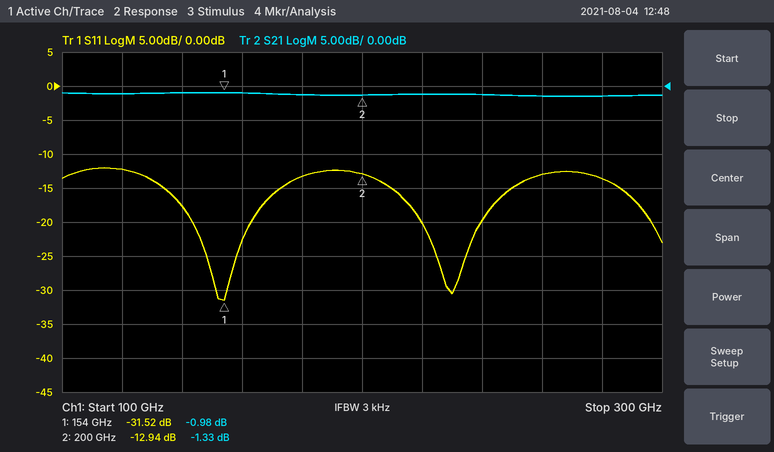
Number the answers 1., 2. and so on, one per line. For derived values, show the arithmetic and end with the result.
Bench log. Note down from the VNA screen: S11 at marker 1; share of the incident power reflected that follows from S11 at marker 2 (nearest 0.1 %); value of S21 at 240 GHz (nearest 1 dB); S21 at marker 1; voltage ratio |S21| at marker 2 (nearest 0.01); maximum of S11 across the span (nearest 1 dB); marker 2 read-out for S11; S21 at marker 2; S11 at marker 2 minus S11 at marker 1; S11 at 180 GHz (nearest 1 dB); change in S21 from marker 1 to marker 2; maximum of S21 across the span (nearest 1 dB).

1. -31.52 dB
2. 10^(-12.94/10) ≈ 5.1 %
3. -1 dB
4. -0.98 dB
5. 10^(-1.33/20) ≈ 0.86
6. -12 dB
7. -12.94 dB
8. -1.33 dB
9. -12.94 − (-31.52) = 18.58 dB
10. -13 dB
11. -1.33 − (-0.98) = -0.35 dB
12. -1 dB
